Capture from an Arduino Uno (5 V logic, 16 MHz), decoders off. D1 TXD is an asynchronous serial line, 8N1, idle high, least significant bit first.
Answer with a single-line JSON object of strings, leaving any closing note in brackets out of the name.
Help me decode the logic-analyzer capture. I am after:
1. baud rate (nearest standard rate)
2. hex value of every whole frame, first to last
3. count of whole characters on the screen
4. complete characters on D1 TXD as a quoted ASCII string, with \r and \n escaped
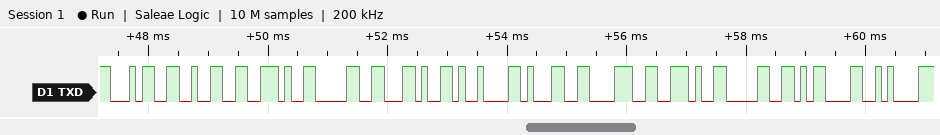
{"baud rate": "9600 baud", "hex value of every whole frame, first to last": "34 32 2E 30 2C 09 31 38 2E 30 0D 0A", "count of whole characters on the screen": "12", "complete characters on D1 TXD as a quoted ASCII string, with \\r and \\n escaped": "\"42.0,\\t18.0\\r\\n\""}
